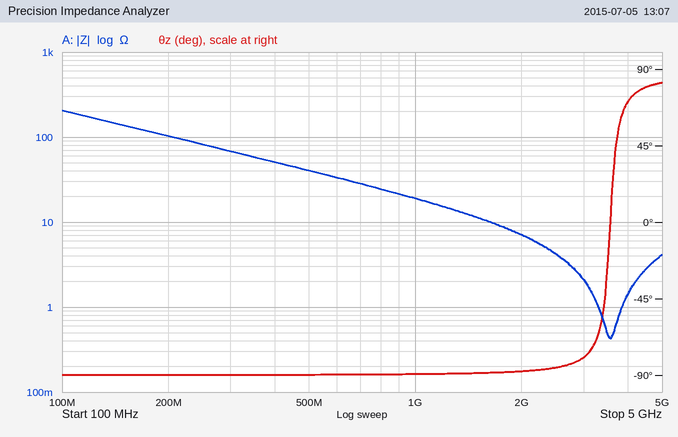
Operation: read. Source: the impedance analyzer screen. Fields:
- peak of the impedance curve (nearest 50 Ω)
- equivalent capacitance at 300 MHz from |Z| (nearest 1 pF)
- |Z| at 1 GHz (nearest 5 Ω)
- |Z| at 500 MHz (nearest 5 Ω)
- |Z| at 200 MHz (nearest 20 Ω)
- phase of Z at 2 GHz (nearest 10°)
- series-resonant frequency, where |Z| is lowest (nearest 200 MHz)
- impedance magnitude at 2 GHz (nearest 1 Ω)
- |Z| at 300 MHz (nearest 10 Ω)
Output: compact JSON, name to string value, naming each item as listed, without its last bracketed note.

{"peak of the impedance curve": "200 Ω", "equivalent capacitance at 300 MHz from |Z|": "8 pF", "|Z| at 1 GHz": "20 Ω", "|Z| at 500 MHz": "40 Ω", "|Z| at 200 MHz": "100 Ω", "phase of Z at 2 GHz": "-90°", "series-resonant frequency, where |Z| is lowest": "3.6 GHz", "impedance magnitude at 2 GHz": "7 Ω", "|Z| at 300 MHz": "70 Ω"}
